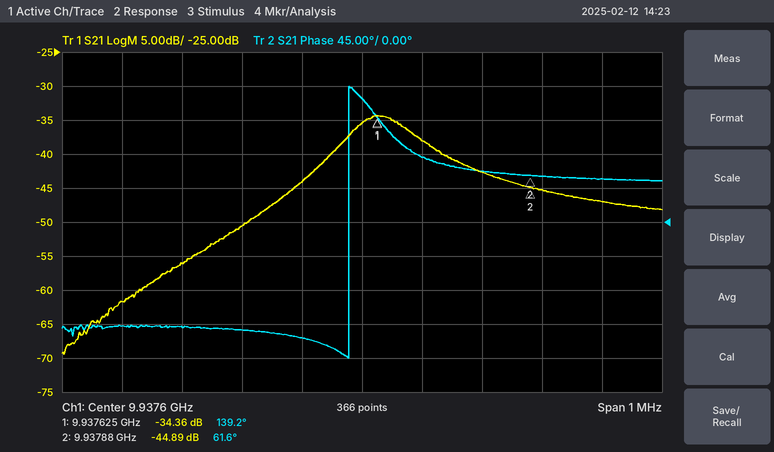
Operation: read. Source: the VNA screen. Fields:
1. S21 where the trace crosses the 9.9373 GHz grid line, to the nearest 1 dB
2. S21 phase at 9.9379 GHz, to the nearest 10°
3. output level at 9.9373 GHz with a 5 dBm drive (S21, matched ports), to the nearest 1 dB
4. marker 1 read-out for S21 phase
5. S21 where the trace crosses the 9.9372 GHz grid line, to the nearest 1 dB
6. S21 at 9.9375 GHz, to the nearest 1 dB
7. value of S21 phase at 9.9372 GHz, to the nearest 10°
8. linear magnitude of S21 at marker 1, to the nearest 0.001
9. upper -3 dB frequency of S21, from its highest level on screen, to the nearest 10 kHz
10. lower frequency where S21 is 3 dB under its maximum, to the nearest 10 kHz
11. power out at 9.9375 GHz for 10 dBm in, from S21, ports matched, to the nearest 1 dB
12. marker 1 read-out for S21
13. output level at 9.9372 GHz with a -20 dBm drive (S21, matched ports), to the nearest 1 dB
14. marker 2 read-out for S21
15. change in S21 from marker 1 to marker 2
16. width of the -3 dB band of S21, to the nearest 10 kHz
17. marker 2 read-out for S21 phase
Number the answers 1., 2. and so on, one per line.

1. -56 dB
2. 60°
3. -51 dBm
4. 139.2°
5. -62 dB
6. -44 dB
7. -140°
8. 0.019
9. 9.93769 GHz
10. 9.93758 GHz
11. -34 dBm
12. -34.36 dB
13. -82 dBm
14. -44.89 dB
15. -10.53 dB
16. 110 kHz
17. 61.6°
